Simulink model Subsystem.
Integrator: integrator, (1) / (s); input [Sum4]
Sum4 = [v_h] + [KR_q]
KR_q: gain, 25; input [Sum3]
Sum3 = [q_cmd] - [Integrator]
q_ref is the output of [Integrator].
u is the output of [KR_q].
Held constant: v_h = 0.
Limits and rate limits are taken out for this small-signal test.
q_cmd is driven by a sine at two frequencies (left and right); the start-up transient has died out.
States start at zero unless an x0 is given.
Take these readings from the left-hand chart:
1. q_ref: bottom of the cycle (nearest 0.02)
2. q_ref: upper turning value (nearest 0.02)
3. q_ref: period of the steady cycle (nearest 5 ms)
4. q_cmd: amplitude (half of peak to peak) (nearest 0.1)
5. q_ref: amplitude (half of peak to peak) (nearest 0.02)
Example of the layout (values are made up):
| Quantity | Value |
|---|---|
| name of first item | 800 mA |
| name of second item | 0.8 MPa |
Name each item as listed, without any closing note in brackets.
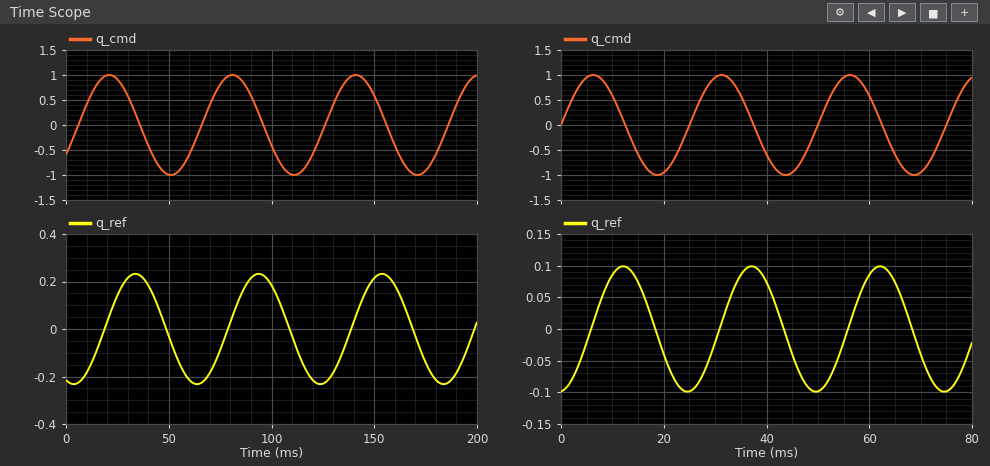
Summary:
| Quantity | Value |
|---|---|
| q_ref: bottom of the cycle | -0.24 |
| q_ref: upper turning value | 0.24 |
| q_ref: period of the steady cycle | 60 ms |
| q_cmd: amplitude (half of peak to peak) | 1.0 |
| q_ref: amplitude (half of peak to peak) | 0.24 |
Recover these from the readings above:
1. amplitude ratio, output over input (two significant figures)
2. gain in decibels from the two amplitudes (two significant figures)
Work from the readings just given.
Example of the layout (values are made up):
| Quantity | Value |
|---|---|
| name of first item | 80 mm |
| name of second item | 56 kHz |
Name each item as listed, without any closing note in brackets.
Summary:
| Quantity | Value |
|---|---|
| amplitude ratio, output over input | 0.24 |
| gain in decibels from the two amplitudes | -12 dB |
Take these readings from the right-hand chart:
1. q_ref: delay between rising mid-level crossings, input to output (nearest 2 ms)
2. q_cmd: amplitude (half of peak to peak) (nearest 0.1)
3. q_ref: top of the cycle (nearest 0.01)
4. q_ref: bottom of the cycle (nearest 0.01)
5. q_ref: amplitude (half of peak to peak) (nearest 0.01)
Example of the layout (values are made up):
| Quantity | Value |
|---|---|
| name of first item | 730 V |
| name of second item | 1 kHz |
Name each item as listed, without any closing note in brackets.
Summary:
| Quantity | Value |
|---|---|
| q_ref: delay between rising mid-level crossings, input to output | 6 ms |
| q_cmd: amplitude (half of peak to peak) | 1.0 |
| q_ref: top of the cycle | 0.10 |
| q_ref: bottom of the cycle | -0.10 |
| q_ref: amplitude (half of peak to peak) | 0.10 |
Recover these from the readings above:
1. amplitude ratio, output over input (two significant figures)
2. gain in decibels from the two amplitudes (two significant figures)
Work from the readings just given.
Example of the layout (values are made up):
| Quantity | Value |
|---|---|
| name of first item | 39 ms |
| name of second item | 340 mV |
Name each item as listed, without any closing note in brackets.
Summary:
| Quantity | Value |
|---|---|
| amplitude ratio, output over input | 0.10 |
| gain in decibels from the two amplitudes | -20 dB |
